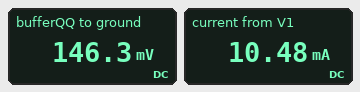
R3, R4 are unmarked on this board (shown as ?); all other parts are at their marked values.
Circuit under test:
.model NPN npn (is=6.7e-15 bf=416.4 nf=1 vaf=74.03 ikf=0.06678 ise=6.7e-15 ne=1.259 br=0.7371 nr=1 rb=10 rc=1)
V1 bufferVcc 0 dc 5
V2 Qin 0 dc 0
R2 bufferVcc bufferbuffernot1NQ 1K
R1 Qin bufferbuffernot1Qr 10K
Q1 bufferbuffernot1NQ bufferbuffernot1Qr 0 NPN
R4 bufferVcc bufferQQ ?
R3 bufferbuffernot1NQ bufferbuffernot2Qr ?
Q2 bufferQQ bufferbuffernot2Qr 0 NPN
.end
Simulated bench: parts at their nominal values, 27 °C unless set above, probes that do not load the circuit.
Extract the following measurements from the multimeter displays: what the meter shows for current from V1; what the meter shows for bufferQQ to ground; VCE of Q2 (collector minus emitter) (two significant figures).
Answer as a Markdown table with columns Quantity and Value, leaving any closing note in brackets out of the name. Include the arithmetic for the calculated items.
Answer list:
| Quantity | Value |
|---|---|
| what the meter shows for current from V1 | 10.48 mA |
| what the meter shows for bufferQQ to ground | 146.3 mV |
| VCE of Q2 (collector minus emitter) | 146.3 mV = 150 mV |
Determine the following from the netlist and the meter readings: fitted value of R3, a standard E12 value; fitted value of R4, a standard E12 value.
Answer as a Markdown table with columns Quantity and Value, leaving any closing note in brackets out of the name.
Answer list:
| Quantity | Value |
|---|---|
| fitted value of R3, a standard E12 value | 27 kΩ |
| fitted value of R4, a standard E12 value | 470 Ω |
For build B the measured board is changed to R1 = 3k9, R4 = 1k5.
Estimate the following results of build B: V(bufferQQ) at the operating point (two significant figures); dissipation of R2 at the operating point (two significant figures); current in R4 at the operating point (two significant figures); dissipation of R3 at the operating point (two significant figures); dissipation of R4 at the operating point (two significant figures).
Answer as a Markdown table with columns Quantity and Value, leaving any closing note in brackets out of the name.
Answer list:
| Quantity | Value |
|---|---|
| V(bufferQQ) at the operating point | 98 mV |
| dissipation of R2 at the operating point | 24 µW |
| current in R4 at the operating point | 3.3 mA |
| dissipation of R3 at the operating point | 640 µW |
| dissipation of R4 at the operating point | 16 mW |
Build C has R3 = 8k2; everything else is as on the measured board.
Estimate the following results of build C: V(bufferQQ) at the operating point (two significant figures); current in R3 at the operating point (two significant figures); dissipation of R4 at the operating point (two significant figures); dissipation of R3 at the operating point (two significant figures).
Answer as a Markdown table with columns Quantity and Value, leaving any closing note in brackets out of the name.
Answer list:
| Quantity | Value |
|---|---|
| V(bufferQQ) at the operating point | 110 mV |
| current in R3 at the operating point | 460 µA |
| dissipation of R4 at the operating point | 51 mW |
| dissipation of R3 at the operating point | 1.8 mW |
